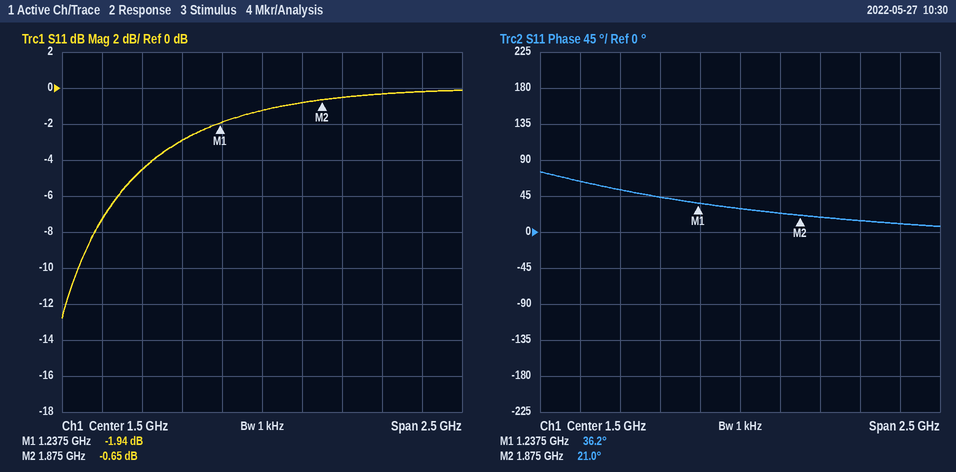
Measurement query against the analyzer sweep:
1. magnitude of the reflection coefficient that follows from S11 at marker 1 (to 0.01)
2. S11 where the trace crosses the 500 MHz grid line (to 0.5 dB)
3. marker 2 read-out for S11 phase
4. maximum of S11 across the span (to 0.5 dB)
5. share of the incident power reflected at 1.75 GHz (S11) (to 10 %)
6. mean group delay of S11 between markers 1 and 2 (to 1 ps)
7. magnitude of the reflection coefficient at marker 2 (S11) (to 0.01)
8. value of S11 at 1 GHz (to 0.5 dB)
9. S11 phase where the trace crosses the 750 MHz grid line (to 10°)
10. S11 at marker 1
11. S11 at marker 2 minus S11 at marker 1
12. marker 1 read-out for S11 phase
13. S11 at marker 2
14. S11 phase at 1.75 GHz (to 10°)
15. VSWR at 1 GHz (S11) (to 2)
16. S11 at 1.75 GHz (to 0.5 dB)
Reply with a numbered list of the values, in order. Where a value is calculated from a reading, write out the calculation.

1. 10^(-1.94/20) ≈ 0.80
2. -7.5 dB
3. 21.0°
4. 0.0 dB
5. 10^(-1/10) ≈ 79.4 %, so 80 % to the nearest 10 %
6. −(21° − (36.2°))/(360° × 637.5 MHz) ≈ 66 ps
7. 10^(-0.65/20) ≈ 0.93
8. -3.0 dB
9. 50°
10. -1.94 dB
11. -0.65 − (-1.94) = 1.29 dB
12. 36.2°
13. -0.65 dB
14. 20°
15. |Γ| = 10^(-3/20) = 0.7079; VSWR = (1 + 0.7079)/(1 − 0.7079) ≈ 6
16. -1.0 dB
